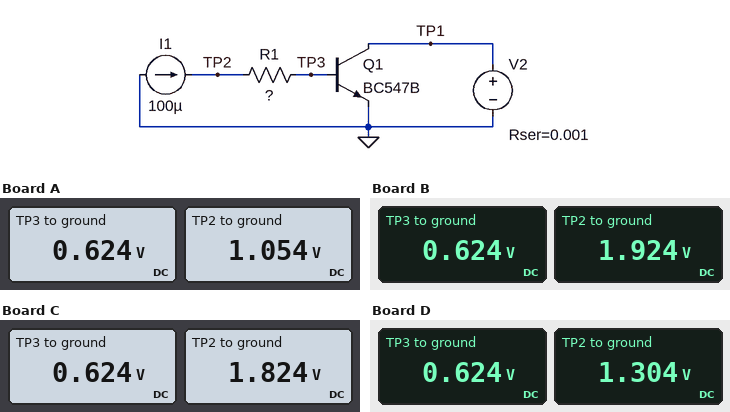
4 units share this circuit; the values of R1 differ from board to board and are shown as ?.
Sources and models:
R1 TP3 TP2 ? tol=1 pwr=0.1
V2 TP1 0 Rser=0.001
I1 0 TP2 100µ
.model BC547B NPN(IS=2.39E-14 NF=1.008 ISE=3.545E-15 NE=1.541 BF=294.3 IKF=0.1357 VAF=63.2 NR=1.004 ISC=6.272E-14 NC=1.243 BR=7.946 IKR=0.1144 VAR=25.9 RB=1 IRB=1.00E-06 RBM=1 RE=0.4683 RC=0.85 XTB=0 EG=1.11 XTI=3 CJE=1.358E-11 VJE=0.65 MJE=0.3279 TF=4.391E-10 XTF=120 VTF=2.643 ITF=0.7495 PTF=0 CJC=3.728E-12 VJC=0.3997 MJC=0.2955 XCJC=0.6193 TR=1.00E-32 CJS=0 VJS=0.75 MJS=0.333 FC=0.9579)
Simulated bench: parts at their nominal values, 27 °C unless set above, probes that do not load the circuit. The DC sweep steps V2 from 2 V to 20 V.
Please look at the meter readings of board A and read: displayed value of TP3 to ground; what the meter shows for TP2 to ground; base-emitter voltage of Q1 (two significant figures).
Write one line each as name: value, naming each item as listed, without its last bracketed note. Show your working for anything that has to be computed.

displayed value of TP3 to ground: 0.624 V
what the meter shows for TP2 to ground: 1.054 V
base-emitter voltage of Q1: 624 mV = 620 mV
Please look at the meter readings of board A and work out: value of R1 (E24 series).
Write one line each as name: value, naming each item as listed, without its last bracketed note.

value of R1: 4.3 kΩ
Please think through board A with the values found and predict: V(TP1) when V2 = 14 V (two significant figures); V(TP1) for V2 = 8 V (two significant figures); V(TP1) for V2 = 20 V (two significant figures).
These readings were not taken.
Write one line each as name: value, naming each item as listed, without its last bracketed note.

V(TP1) when V2 = 14 V: 14 V
V(TP1) for V2 = 8 V: 8.0 V
V(TP1) for V2 = 20 V: 20 V
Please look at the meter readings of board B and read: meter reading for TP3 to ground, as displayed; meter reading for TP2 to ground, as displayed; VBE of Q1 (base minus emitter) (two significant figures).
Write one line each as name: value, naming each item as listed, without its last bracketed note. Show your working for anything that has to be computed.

meter reading for TP3 to ground, as displayed: 0.624 V
meter reading for TP2 to ground, as displayed: 1.924 V
VBE of Q1 (base minus emitter): 624 mV = 620 mV
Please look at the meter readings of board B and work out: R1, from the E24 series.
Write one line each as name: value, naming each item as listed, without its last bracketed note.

R1, from the E24 series: 13 kΩ
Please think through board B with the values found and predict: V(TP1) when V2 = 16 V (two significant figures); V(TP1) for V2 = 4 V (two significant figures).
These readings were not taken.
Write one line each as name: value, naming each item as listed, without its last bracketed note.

V(TP1) when V2 = 16 V: 16 V
V(TP1) for V2 = 4 V: 4.0 V
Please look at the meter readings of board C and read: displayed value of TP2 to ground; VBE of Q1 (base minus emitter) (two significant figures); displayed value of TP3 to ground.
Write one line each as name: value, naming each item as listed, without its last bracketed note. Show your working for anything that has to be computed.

displayed value of TP2 to ground: 1.824 V
VBE of Q1 (base minus emitter): 624 mV = 620 mV
displayed value of TP3 to ground: 0.624 V
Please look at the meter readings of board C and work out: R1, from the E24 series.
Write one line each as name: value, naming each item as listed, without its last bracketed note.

R1, from the E24 series: 12 kΩ
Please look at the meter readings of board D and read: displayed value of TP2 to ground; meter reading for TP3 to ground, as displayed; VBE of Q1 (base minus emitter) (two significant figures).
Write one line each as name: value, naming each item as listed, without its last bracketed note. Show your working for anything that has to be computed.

displayed value of TP2 to ground: 1.304 V
meter reading for TP3 to ground, as displayed: 0.624 V
VBE of Q1 (base minus emitter): 624 mV = 620 mV
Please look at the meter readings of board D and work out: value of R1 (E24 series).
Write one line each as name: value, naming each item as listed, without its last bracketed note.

value of R1: 6.8 kΩ
